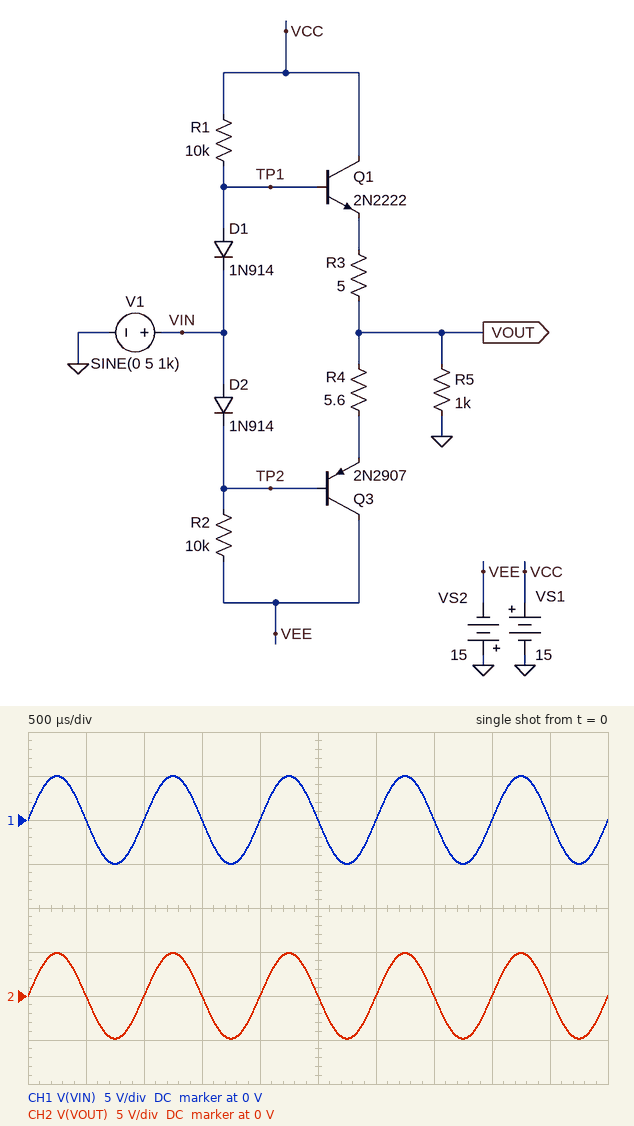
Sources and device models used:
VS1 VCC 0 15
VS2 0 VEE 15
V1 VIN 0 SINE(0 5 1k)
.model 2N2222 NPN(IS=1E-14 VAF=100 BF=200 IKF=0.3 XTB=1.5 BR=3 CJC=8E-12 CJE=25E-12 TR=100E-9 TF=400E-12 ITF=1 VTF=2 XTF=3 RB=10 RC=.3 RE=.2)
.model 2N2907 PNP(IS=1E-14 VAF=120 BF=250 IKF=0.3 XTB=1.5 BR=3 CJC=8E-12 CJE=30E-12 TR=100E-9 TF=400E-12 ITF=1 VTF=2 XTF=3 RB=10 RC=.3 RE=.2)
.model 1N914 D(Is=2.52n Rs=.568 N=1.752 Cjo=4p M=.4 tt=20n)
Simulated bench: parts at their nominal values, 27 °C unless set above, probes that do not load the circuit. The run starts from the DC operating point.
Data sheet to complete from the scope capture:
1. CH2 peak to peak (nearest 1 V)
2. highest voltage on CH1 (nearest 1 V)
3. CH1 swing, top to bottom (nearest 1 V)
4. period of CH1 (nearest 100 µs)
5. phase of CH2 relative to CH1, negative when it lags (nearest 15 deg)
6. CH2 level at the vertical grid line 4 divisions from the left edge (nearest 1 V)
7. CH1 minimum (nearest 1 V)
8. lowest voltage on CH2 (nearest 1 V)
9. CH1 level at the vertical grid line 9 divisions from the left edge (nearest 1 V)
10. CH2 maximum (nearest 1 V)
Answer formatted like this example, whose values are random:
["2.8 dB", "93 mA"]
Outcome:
["10 V", "5 V", "10 V", "1.0 ms", "0 deg", "0 V", "-5 V", "-5 V", "0 V", "5 V"]
